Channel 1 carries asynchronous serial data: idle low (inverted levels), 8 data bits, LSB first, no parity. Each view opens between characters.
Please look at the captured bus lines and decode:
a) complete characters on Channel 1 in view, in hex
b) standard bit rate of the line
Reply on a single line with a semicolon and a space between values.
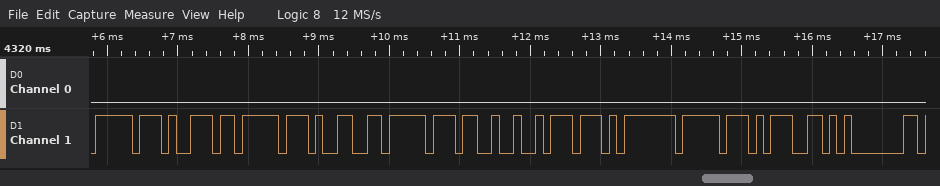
10, 23, 10, 33, 10, B6, 11, 01, 10, 31, FD; 9600 baud
